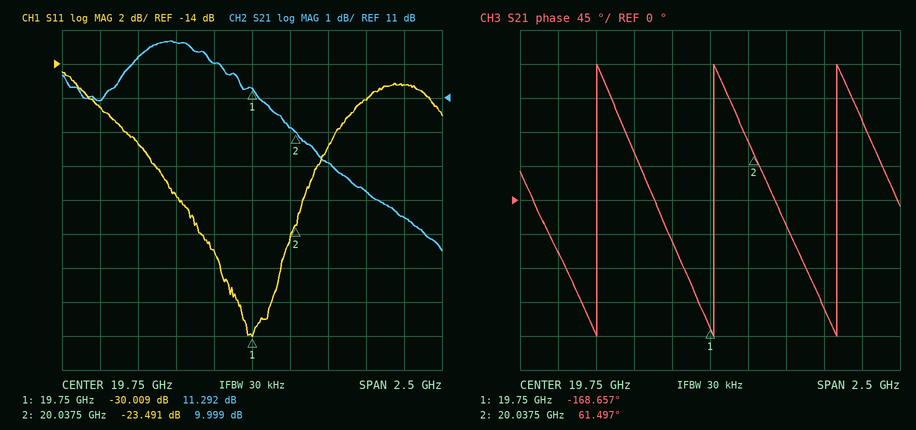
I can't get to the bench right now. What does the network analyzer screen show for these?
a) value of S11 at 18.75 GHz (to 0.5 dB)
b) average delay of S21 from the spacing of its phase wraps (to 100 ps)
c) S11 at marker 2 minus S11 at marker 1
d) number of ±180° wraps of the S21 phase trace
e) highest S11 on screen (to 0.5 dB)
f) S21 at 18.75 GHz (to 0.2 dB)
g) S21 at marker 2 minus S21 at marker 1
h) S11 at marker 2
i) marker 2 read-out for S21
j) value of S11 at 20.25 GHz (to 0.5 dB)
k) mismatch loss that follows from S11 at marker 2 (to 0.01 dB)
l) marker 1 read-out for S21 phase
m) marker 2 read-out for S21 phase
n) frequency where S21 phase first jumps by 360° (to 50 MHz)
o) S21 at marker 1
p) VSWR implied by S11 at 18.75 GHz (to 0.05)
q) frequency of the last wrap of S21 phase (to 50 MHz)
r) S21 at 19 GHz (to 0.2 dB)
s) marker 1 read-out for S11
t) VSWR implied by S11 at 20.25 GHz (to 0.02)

-16.5 dB
1.3 ns
6.518 dB
3
-14.5 dB
11.0 dB
-1.293 dB
-23.491 dB
9.999 dB
-19.0 dB
0.02 dB
-168.657°
61.497°
19.00 GHz
11.292 dB
1.35
20.60 GHz
12.2 dB
-30.009 dB
1.26
